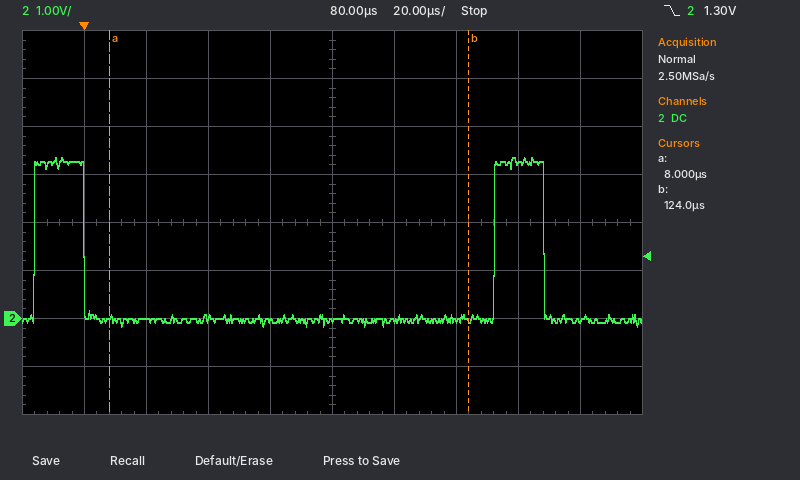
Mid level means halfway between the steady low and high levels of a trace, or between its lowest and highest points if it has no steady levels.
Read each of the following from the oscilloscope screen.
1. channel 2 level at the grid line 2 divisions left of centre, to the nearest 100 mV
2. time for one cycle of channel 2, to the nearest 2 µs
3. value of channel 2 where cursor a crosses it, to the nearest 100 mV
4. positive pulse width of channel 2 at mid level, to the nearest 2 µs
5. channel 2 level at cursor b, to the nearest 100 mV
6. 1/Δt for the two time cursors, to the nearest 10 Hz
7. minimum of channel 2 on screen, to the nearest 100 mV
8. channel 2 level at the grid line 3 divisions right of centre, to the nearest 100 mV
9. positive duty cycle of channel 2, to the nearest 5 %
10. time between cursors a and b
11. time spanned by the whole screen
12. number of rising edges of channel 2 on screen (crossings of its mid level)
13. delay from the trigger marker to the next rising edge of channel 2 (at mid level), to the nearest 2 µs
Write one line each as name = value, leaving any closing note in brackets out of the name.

channel 2 level at the grid line 2 divisions left of centre, to the nearest 100 mV = 0.0 V
time for one cycle of channel 2, to the nearest 2 µs = 148 µs
value of channel 2 where cursor a crosses it, to the nearest 100 mV = 0.0 V
positive pulse width of channel 2 at mid level, to the nearest 2 µs = 16 µs
channel 2 level at cursor b, to the nearest 100 mV = 0.0 V
1/Δt for the two time cursors, to the nearest 10 Hz = 8.62 kHz
minimum of channel 2 on screen, to the nearest 100 mV = -200 mV
channel 2 level at the grid line 3 divisions right of centre, to the nearest 100 mV = 3.3 V
positive duty cycle of channel 2, to the nearest 5 % = 10 %
time between cursors a and b = 116 µs
time spanned by the whole screen = 200 µs
number of rising edges of channel 2 on screen = 2
delay from the trigger marker to the next rising edge of channel 2 (at mid level), to the nearest 2 µs = 132 µs
